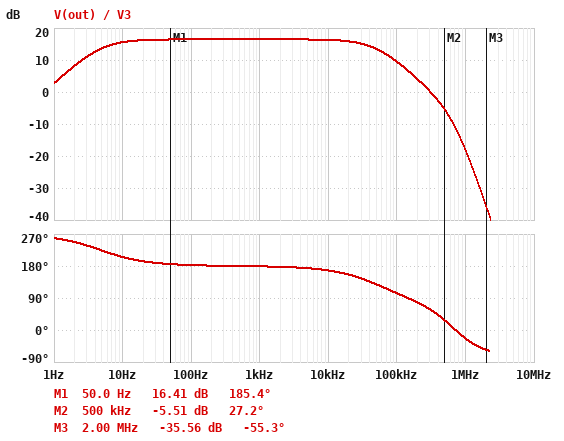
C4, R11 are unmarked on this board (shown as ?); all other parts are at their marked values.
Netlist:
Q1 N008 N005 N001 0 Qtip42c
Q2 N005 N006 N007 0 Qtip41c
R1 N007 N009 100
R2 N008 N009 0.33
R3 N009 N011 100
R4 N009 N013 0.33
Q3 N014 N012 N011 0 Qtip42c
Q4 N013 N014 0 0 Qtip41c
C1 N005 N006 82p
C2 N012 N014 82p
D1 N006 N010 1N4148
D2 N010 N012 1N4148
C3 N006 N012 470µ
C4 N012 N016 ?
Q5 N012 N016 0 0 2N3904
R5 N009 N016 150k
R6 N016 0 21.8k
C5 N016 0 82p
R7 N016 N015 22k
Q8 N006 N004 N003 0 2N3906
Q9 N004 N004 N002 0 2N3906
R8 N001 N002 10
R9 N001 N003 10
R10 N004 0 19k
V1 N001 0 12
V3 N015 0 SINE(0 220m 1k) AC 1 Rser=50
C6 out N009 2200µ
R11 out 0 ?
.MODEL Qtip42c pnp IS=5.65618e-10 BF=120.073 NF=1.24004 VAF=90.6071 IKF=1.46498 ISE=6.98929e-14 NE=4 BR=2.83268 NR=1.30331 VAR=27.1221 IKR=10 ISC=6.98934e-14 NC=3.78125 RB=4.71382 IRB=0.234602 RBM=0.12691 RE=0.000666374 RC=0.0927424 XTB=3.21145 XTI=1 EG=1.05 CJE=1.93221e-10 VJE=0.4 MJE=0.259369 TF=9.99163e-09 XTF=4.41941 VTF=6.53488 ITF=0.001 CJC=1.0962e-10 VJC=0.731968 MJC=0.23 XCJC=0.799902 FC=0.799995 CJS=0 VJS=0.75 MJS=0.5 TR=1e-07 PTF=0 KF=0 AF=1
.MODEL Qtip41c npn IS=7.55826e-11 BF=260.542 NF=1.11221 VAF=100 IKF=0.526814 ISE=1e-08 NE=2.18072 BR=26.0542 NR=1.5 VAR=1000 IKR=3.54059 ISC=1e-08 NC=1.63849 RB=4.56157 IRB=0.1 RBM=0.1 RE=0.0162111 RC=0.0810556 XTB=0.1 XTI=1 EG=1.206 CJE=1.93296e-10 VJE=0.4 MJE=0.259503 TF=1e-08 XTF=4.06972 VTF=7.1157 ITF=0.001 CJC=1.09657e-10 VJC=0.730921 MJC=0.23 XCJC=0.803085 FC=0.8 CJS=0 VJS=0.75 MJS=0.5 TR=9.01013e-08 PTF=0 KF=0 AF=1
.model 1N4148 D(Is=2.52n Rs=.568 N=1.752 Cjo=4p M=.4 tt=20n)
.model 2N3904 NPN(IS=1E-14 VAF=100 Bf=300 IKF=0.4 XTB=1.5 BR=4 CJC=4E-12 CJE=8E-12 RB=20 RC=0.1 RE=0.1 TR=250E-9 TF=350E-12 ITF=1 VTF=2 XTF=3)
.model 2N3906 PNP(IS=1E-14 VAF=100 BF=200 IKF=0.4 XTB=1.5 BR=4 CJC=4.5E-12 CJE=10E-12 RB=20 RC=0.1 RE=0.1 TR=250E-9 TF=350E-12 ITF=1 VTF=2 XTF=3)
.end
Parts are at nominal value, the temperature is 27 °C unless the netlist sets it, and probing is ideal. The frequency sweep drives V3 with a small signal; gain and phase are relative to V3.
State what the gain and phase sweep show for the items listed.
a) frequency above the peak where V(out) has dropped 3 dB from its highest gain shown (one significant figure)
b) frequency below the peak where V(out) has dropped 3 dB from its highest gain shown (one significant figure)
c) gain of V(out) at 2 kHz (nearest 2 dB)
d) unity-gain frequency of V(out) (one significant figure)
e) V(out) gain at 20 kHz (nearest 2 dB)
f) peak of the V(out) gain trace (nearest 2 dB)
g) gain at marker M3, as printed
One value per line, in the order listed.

50 kHz
5 Hz
16 dB
300 kHz
16 dB
16 dB
-35.56 dB
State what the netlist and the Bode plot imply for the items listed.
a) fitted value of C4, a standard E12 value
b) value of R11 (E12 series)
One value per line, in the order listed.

18 pF
15 Ω
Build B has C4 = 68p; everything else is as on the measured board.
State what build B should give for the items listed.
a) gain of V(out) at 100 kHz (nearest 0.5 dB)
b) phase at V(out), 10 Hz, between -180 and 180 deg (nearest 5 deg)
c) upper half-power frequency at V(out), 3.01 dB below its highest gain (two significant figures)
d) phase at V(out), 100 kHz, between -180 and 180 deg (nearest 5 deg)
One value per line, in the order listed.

-0.5 dB
-155 deg
15 kHz
90 deg
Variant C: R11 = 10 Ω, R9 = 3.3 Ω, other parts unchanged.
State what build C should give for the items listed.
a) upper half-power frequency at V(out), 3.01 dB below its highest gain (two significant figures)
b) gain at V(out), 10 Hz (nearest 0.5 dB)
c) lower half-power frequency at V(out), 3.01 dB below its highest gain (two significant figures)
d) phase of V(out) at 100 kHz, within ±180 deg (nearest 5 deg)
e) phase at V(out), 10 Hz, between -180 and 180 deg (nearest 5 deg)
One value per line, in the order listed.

51 kHz
14.5 dB
7.1 Hz
100 deg
-145 deg
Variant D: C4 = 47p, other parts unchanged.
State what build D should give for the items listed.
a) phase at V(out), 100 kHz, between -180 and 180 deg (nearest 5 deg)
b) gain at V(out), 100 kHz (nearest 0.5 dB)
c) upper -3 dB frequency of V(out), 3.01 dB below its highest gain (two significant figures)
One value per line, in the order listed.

90 deg
2.5 dB
21 kHz
